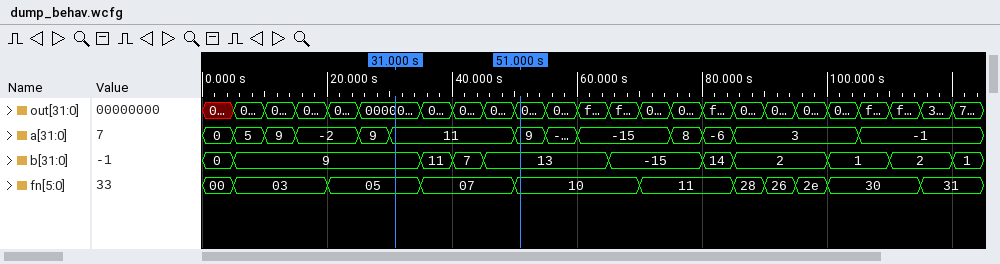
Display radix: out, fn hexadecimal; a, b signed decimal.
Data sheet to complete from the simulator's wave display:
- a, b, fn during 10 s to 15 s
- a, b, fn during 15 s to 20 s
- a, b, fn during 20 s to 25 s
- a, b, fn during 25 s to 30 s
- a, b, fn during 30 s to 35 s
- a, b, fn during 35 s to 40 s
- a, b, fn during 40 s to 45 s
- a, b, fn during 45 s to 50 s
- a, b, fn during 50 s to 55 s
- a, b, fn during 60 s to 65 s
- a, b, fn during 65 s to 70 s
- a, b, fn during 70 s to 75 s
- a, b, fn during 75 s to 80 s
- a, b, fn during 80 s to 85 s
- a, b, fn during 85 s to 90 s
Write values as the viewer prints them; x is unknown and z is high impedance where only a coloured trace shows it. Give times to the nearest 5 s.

a=9, b=9, fn=03
a=-2, b=9, fn=03
a=-2, b=9, fn=05
a=9, b=9, fn=05
a=11, b=9, fn=05
a=11, b=11, fn=07
a=11, b=7, fn=07
a=11, b=13, fn=07
a=9, b=13, fn=10
a=-15, b=13, fn=10
a=-15, b=-15, fn=10
a=-15, b=-15, fn=11
a=8, b=-15, fn=11
a=-6, b=14, fn=11
a=3, b=2, fn=28
